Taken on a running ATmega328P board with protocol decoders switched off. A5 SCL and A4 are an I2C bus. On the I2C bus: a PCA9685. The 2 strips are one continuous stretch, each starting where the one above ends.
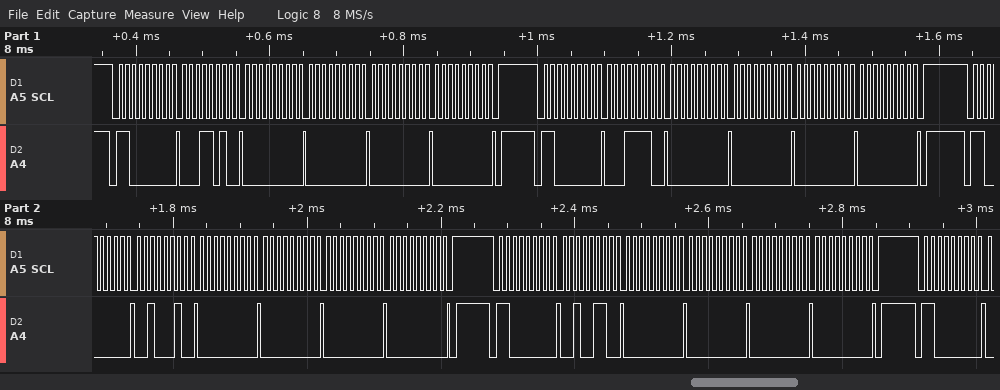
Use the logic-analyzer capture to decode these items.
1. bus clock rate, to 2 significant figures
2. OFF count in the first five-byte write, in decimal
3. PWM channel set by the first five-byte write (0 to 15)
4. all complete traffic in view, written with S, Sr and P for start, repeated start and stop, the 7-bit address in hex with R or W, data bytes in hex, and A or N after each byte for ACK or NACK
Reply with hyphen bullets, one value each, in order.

- 100 kHz
- 0
- 5
- S 60W A 1A A 00 A 00 A 00 A 00 A P S 60W A 1E A 00 A 00 A 00 A 00 A P S 60W A 22 A 00 A 00 A 00 A 00 A P S 60W A 26 A 00 A 00 A 00 A 00 A P S 60W A
